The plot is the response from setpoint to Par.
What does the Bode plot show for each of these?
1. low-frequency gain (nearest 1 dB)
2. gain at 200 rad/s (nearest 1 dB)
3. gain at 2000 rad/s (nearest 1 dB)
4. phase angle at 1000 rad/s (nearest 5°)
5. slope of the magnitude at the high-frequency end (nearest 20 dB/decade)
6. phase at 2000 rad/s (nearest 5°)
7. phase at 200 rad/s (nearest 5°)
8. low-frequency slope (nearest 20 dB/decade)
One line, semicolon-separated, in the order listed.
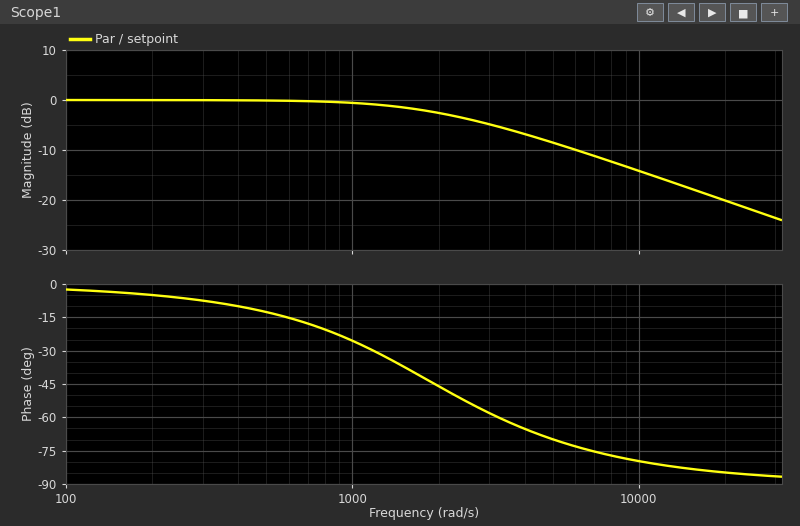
0 dB; 0 dB; -3 dB; -25°; -20 dB/decade; -45°; -5°; 0 dB/decade
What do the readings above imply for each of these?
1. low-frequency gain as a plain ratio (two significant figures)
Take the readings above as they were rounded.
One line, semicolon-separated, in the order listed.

1.0
